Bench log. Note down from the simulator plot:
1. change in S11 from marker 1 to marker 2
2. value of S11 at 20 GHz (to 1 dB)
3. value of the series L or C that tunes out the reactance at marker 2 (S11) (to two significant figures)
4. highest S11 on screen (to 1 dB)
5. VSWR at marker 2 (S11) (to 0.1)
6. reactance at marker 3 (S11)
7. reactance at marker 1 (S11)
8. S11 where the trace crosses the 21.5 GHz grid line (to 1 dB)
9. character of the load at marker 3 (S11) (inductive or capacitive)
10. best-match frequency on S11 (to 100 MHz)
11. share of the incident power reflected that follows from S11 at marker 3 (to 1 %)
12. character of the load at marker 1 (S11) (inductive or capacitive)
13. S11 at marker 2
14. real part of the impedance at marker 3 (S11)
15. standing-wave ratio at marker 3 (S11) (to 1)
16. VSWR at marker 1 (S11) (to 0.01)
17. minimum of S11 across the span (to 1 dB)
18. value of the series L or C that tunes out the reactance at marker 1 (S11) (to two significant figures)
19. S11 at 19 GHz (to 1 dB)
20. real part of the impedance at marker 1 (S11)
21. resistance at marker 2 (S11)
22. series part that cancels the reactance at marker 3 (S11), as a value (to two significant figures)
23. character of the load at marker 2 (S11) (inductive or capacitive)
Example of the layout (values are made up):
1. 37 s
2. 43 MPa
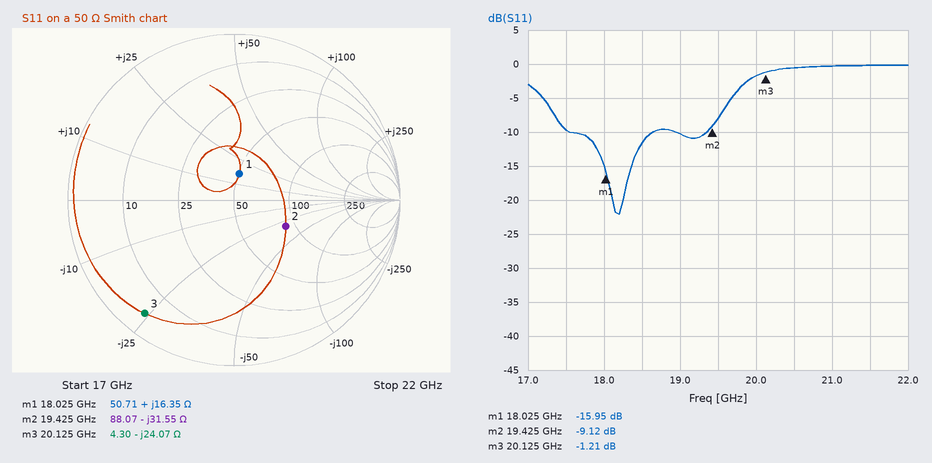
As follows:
1. 6.83 dB
2. -2 dB
3. 260 pH
4. 0 dB
5. 2.1
6. -24.07 Ω
7. +16.35 Ω
8. 0 dB
9. capacitive
10. 18.2 GHz
11. 76 %
12. inductive
13. -9.12 dB
14. 4.30 Ω
15. 14
16. 1.38
17. -22 dB
18. 540 fF
19. -10 dB
20. 50.71 Ω
21. 88.07 Ω
22. 190 pH
23. capacitive
